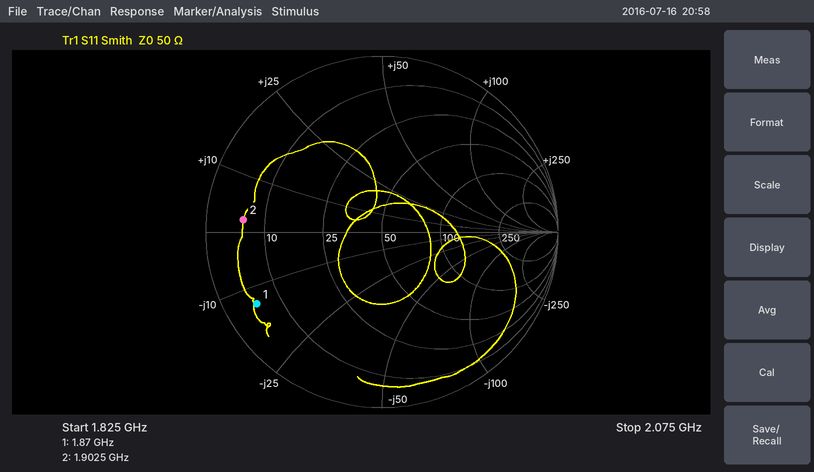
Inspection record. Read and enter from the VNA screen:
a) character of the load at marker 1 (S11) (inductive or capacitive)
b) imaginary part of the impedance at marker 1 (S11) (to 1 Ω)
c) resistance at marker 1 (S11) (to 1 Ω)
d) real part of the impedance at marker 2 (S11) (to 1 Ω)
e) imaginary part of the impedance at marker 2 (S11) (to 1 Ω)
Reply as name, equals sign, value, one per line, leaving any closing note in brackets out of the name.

character of the load at marker 1 (S11) = capacitive
imaginary part of the impedance at marker 1 (S11) = -13 Ω
resistance at marker 1 (S11) = 5 Ω
real part of the impedance at marker 2 (S11) = 6 Ω
imaginary part of the impedance at marker 2 (S11) = +2 Ω
